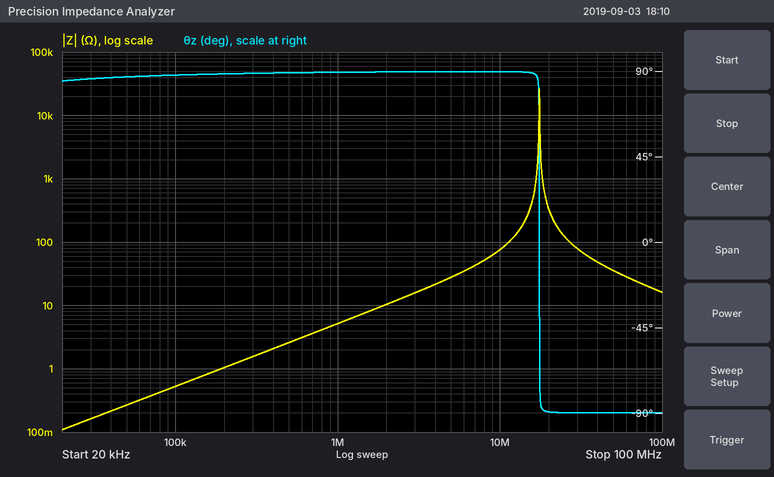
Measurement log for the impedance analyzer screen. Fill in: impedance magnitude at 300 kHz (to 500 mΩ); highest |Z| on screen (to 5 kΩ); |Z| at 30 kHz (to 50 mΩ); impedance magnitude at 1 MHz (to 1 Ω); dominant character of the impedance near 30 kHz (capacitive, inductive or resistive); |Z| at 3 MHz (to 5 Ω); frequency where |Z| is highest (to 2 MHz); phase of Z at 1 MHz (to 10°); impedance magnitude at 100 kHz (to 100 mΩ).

1.5 Ω
25 kΩ
150 mΩ
5 Ω
inductive
15 Ω
18 MHz
90°
500 mΩ
